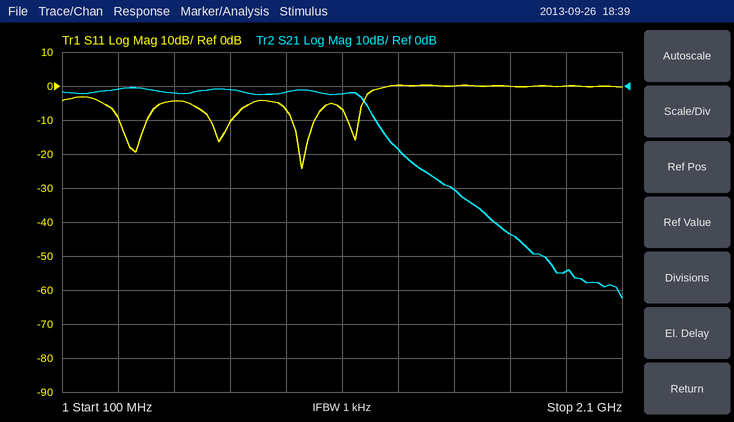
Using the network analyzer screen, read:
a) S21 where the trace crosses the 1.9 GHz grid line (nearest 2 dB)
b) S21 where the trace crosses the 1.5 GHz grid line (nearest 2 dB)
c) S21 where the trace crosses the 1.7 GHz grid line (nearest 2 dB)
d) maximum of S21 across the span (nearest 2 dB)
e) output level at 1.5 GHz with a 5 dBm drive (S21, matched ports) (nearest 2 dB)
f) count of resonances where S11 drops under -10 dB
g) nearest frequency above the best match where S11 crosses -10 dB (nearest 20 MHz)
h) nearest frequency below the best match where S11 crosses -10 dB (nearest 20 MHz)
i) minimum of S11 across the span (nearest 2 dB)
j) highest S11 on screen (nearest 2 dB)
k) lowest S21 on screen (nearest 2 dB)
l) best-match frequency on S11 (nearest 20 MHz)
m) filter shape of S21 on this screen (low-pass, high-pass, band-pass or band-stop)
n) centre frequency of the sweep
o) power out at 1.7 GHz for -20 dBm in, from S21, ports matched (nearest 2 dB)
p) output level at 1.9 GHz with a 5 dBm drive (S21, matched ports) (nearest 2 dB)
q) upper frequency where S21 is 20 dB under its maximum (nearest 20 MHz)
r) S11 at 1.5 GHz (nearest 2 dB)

-54 dB
-30 dB
-44 dB
0 dB
-26 dBm
4
1.00 GHz
920 MHz
-24 dB
0 dB
-62 dB
960 MHz
low-pass
1.1 GHz
-64 dBm
-50 dBm
1.32 GHz
0 dB
